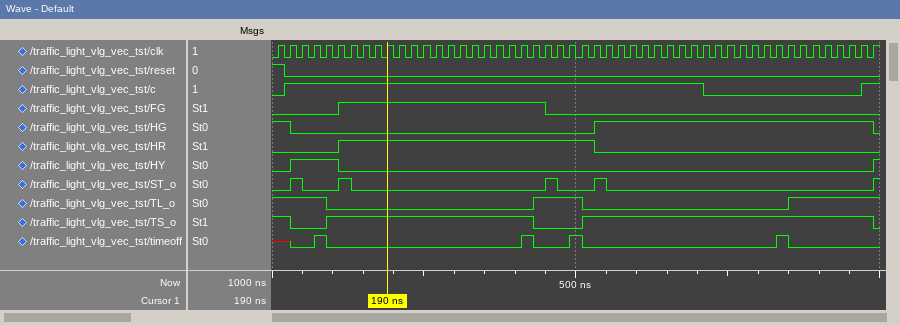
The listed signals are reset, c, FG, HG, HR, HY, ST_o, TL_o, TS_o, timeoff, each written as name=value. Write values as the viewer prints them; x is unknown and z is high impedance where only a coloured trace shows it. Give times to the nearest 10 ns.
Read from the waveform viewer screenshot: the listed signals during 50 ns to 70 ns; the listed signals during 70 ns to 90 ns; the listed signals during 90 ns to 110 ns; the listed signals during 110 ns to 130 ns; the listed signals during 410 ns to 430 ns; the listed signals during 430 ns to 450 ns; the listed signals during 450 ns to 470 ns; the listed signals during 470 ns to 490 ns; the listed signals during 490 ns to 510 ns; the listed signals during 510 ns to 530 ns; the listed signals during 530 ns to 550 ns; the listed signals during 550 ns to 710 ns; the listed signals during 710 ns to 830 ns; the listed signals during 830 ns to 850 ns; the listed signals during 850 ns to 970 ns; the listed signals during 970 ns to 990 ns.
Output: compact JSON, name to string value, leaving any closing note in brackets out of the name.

{"the listed signals during 50 ns to 70 ns": "reset=0, c=1, FG=0, HG=0, HR=0, HY=1, ST_o=0, TL_o=1, TS_o=0, timeoff=0", "the listed signals during 70 ns to 90 ns": "reset=0, c=1, FG=0, HG=0, HR=0, HY=1, ST_o=0, TL_o=1, TS_o=0, timeoff=1", "the listed signals during 90 ns to 110 ns": "reset=0, c=1, FG=0, HG=0, HR=0, HY=1, ST_o=0, TL_o=0, TS_o=1, timeoff=0", "the listed signals during 110 ns to 130 ns": "reset=0, c=1, FG=1, HG=0, HR=1, HY=0, ST_o=1, TL_o=0, TS_o=1, timeoff=0", "the listed signals during 410 ns to 430 ns": "reset=0, c=1, FG=1, HG=0, HR=1, HY=0, ST_o=0, TL_o=0, TS_o=1, timeoff=1", "the listed signals during 430 ns to 450 ns": "reset=0, c=1, FG=1, HG=0, HR=1, HY=0, ST_o=0, TL_o=1, TS_o=0, timeoff=0", "the listed signals during 450 ns to 470 ns": "reset=0, c=1, FG=0, HG=0, HR=1, HY=0, ST_o=1, TL_o=1, TS_o=0, timeoff=0", "the listed signals during 470 ns to 490 ns": "reset=0, c=1, FG=0, HG=0, HR=1, HY=0, ST_o=0, TL_o=1, TS_o=0, timeoff=0", "the listed signals during 490 ns to 510 ns": "reset=0, c=1, FG=0, HG=0, HR=1, HY=0, ST_o=0, TL_o=1, TS_o=0, timeoff=1", "the listed signals during 510 ns to 530 ns": "reset=0, c=1, FG=0, HG=0, HR=1, HY=0, ST_o=0, TL_o=0, TS_o=1, timeoff=0", "the listed signals during 530 ns to 550 ns": "reset=0, c=1, FG=0, HG=1, HR=0, HY=0, ST_o=1, TL_o=0, TS_o=1, timeoff=0", "the listed signals during 550 ns to 710 ns": "reset=0, c=1, FG=0, HG=1, HR=0, HY=0, ST_o=0, TL_o=0, TS_o=1, timeoff=0", "the listed signals during 710 ns to 830 ns": "reset=0, c=0, FG=0, HG=1, HR=0, HY=0, ST_o=0, TL_o=0, TS_o=1, timeoff=0", "the listed signals during 830 ns to 850 ns": "reset=0, c=0, FG=0, HG=1, HR=0, HY=0, ST_o=0, TL_o=0, TS_o=1, timeoff=1", "the listed signals during 850 ns to 970 ns": "reset=0, c=0, FG=0, HG=1, HR=0, HY=0, ST_o=0, TL_o=1, TS_o=1, timeoff=0", "the listed signals during 970 ns to 990 ns": "reset=0, c=1, FG=0, HG=1, HR=0, HY=0, ST_o=0, TL_o=1, TS_o=1, timeoff=0"}
